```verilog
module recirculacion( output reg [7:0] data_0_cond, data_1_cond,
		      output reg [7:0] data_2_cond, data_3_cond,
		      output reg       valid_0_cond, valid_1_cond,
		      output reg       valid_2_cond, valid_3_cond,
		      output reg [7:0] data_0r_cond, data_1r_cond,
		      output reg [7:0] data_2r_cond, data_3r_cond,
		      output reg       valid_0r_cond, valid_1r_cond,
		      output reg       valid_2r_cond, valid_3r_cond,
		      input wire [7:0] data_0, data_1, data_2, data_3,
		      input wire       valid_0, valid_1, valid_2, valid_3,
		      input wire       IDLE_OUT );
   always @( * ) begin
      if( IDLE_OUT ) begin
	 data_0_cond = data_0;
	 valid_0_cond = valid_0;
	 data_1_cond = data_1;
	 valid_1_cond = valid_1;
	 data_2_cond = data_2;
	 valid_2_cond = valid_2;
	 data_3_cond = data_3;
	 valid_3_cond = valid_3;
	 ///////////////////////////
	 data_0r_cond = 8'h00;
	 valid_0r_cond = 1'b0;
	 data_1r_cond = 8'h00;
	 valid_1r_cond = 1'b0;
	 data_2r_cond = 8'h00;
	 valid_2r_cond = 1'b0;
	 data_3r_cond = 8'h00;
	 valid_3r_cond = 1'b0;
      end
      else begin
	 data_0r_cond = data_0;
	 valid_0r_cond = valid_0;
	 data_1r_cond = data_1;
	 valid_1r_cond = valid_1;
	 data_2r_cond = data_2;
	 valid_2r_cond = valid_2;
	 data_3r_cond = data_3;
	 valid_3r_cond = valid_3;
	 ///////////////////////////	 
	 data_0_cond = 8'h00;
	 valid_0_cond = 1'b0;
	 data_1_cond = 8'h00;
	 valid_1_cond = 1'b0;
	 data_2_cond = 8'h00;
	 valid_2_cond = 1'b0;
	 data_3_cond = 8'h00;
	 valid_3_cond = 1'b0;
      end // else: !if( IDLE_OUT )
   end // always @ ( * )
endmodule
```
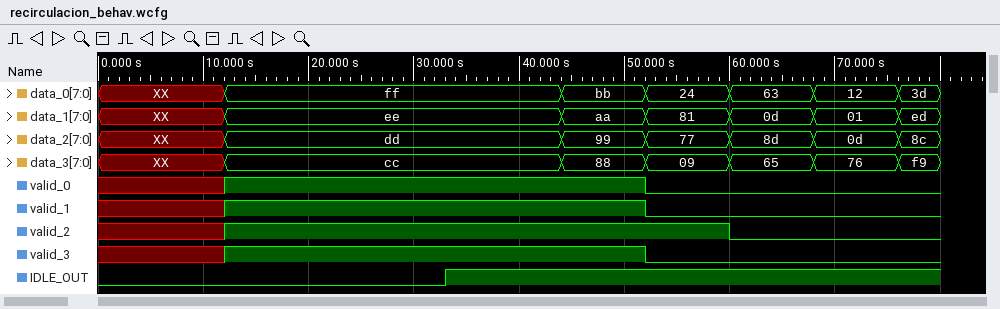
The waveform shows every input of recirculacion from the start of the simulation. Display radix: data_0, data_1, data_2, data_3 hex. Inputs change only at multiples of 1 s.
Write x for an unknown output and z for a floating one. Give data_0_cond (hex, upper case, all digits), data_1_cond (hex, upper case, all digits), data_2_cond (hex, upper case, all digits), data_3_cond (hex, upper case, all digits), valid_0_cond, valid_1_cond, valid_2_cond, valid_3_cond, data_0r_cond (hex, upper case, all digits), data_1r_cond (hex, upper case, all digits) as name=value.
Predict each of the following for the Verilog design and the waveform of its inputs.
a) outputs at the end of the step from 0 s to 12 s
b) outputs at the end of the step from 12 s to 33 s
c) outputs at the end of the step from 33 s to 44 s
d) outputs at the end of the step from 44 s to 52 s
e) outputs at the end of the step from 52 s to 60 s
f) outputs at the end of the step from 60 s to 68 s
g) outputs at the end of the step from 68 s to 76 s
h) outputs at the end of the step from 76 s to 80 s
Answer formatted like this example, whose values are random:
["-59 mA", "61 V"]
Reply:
["data_0_cond=00, data_1_cond=00, data_2_cond=00, data_3_cond=00, valid_0_cond=0, valid_1_cond=0, valid_2_cond=0, valid_3_cond=0, data_0r_cond=x, data_1r_cond=x", "data_0_cond=00, data_1_cond=00, data_2_cond=00, data_3_cond=00, valid_0_cond=0, valid_1_cond=0, valid_2_cond=0, valid_3_cond=0, data_0r_cond=FF, data_1r_cond=EE", "data_0_cond=FF, data_1_cond=EE, data_2_cond=DD, data_3_cond=CC, valid_0_cond=1, valid_1_cond=1, valid_2_cond=1, valid_3_cond=1, data_0r_cond=00, data_1r_cond=00", "data_0_cond=BB, data_1_cond=AA, data_2_cond=99, data_3_cond=88, valid_0_cond=1, valid_1_cond=1, valid_2_cond=1, valid_3_cond=1, data_0r_cond=00, data_1r_cond=00", "data_0_cond=24, data_1_cond=81, data_2_cond=77, data_3_cond=09, valid_0_cond=0, valid_1_cond=0, valid_2_cond=1, valid_3_cond=0, data_0r_cond=00, data_1r_cond=00", "data_0_cond=63, data_1_cond=0D, data_2_cond=8D, data_3_cond=65, valid_0_cond=0, valid_1_cond=0, valid_2_cond=0, valid_3_cond=0, data_0r_cond=00, data_1r_cond=00", "data_0_cond=12, data_1_cond=01, data_2_cond=0D, data_3_cond=76, valid_0_cond=0, valid_1_cond=0, valid_2_cond=0, valid_3_cond=0, data_0r_cond=00, data_1r_cond=00", "data_0_cond=3D, data_1_cond=ED, data_2_cond=8C, data_3_cond=F9, valid_0_cond=0, valid_1_cond=0, valid_2_cond=0, valid_3_cond=0, data_0r_cond=00, data_1r_cond=00"]
